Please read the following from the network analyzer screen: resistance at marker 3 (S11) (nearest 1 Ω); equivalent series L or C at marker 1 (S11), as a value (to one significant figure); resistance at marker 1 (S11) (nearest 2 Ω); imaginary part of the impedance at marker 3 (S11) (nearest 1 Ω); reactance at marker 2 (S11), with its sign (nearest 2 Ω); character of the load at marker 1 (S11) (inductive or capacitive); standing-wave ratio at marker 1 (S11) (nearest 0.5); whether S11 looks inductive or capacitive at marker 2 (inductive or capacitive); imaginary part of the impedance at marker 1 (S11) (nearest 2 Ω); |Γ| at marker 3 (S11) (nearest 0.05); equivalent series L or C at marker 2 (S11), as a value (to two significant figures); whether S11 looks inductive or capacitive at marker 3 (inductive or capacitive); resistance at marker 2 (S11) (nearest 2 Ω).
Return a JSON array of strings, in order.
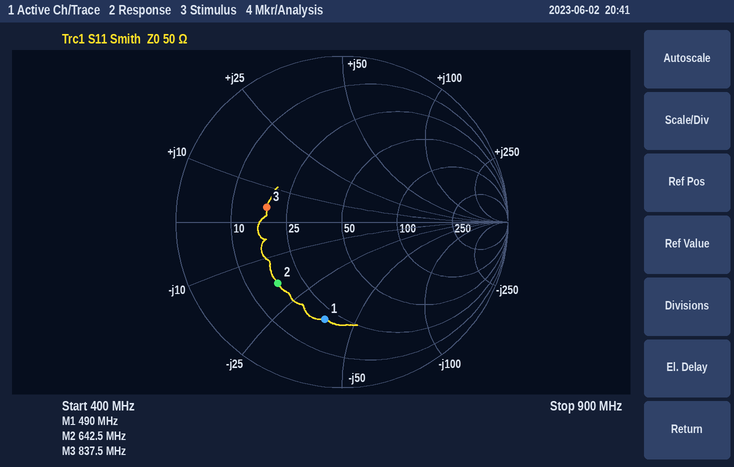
["19 Ω", "9 pF", "20 Ω", "+4 Ω", "-18 Ω", "capacitive", "4.0", "capacitive", "-38 Ω", "0.45", "14 pF", "inductive", "18 Ω"]
